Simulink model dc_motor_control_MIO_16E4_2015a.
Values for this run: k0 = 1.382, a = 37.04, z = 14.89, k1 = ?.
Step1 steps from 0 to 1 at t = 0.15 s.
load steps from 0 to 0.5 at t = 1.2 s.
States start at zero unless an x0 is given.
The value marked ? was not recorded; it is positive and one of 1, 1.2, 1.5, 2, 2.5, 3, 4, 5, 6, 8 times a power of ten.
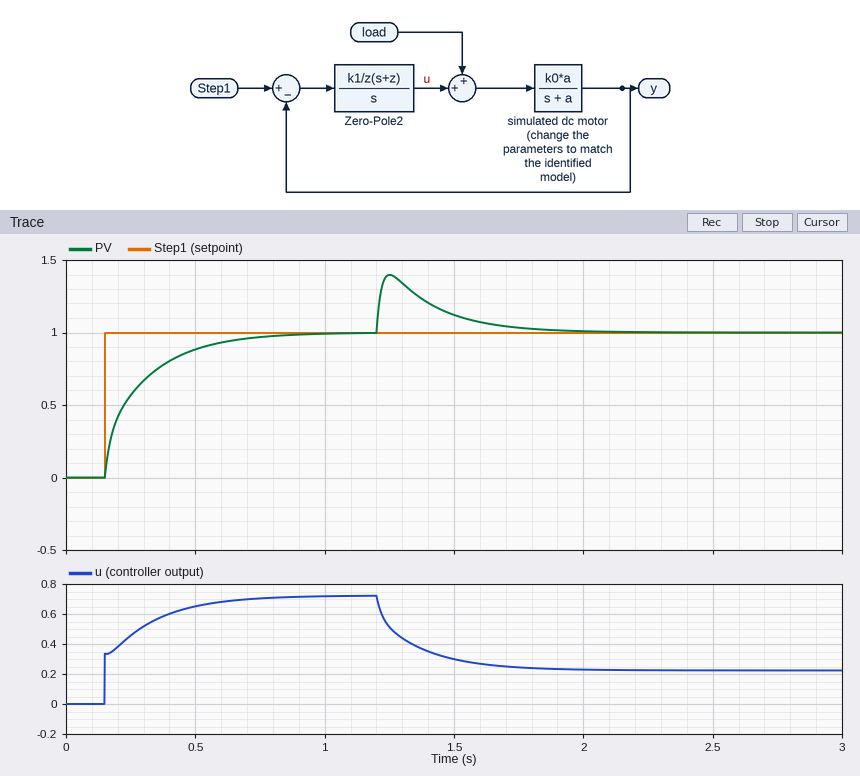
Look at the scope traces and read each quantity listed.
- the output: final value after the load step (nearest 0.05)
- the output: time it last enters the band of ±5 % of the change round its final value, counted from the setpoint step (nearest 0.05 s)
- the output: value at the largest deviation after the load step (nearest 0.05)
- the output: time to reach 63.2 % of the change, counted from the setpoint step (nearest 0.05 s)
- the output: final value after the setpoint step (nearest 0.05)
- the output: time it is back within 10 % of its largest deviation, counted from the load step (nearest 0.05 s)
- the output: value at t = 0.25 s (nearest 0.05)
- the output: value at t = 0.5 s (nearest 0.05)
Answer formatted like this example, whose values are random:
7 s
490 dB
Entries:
1.00
0.50 s
1.40
0.15 s
1.00
0.50 s
0.55
0.90
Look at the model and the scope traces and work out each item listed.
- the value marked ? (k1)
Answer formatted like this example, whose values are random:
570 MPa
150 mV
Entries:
5
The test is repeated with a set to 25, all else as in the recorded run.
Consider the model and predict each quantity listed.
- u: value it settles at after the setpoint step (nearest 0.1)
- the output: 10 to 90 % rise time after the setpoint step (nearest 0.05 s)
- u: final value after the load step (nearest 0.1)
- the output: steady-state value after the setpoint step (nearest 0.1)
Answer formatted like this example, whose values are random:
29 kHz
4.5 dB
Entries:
0.7
0.35 s
0.2
1.0
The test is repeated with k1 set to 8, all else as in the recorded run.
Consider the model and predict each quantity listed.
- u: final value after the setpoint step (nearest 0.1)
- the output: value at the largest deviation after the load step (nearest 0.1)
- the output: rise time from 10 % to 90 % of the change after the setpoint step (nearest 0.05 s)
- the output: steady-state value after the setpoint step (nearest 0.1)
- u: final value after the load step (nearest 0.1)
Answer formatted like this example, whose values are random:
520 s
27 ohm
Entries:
0.7
1.3
0.25 s
1.0
0.2
